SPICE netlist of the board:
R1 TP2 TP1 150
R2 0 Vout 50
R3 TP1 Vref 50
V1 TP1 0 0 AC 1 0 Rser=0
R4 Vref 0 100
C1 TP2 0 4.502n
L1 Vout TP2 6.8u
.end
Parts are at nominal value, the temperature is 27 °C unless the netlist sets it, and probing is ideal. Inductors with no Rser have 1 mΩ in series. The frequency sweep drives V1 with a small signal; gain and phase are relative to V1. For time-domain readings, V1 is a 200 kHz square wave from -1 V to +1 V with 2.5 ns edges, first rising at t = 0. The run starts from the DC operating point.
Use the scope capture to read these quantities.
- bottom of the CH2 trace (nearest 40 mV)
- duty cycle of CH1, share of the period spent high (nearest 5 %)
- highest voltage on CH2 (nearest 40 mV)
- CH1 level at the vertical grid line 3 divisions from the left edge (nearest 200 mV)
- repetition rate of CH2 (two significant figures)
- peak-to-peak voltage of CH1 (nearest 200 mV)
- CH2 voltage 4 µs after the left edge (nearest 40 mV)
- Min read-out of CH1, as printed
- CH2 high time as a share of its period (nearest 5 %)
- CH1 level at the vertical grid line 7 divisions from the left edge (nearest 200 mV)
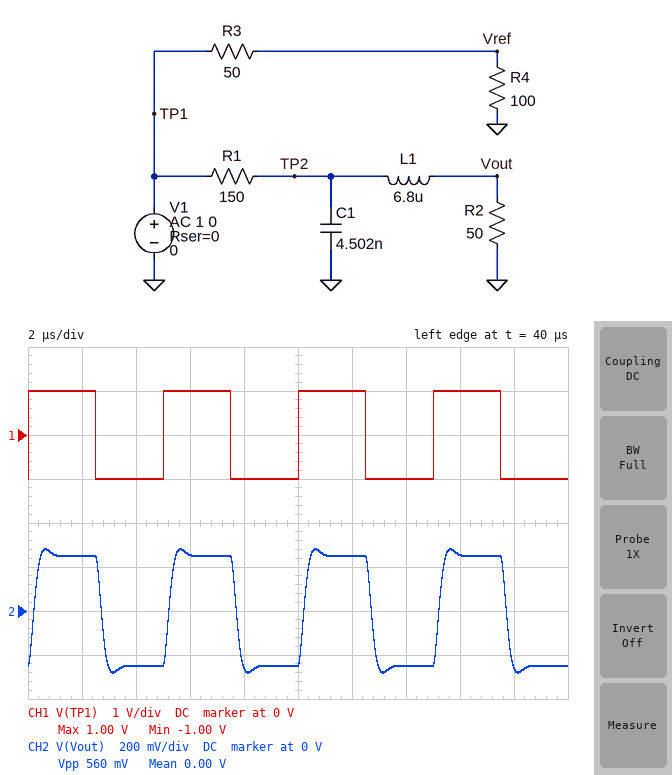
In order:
-280 mV
50 %
280 mV
1.0 V
200 kHz
2.0 V
-240 mV
-1.00 V
50 %
-1.0 V
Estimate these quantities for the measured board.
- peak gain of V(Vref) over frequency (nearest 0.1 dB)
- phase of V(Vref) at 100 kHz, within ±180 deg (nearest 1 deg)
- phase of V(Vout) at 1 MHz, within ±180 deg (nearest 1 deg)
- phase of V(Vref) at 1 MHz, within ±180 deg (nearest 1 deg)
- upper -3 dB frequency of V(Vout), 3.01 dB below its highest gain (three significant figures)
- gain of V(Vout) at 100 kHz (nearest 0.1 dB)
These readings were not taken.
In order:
-3.5 dB
0 deg
-86 deg
0 deg
1.10 MHz
-12.0 dB
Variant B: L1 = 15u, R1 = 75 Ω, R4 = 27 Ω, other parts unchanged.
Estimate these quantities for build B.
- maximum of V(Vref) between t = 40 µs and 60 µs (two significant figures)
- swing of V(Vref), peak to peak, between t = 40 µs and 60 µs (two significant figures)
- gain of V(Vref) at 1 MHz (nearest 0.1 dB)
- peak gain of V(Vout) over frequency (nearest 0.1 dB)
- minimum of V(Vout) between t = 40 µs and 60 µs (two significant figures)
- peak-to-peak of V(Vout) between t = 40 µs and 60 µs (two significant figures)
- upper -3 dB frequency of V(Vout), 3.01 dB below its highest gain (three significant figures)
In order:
350 mV
700 mV
-9.1 dB
-7.8 dB
-460 mV
920 mV
858 kHz
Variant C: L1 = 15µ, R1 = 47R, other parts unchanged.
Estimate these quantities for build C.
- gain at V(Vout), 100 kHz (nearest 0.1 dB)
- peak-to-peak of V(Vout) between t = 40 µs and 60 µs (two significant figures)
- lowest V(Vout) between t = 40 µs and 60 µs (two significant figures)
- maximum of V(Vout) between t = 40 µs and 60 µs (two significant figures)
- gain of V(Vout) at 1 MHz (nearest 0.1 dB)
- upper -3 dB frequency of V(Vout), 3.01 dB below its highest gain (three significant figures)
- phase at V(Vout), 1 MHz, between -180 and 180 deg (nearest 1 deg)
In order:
-5.8 dB
1.1 V
-550 mV
550 mV
-10.3 dB
853 kHz
-100 deg
